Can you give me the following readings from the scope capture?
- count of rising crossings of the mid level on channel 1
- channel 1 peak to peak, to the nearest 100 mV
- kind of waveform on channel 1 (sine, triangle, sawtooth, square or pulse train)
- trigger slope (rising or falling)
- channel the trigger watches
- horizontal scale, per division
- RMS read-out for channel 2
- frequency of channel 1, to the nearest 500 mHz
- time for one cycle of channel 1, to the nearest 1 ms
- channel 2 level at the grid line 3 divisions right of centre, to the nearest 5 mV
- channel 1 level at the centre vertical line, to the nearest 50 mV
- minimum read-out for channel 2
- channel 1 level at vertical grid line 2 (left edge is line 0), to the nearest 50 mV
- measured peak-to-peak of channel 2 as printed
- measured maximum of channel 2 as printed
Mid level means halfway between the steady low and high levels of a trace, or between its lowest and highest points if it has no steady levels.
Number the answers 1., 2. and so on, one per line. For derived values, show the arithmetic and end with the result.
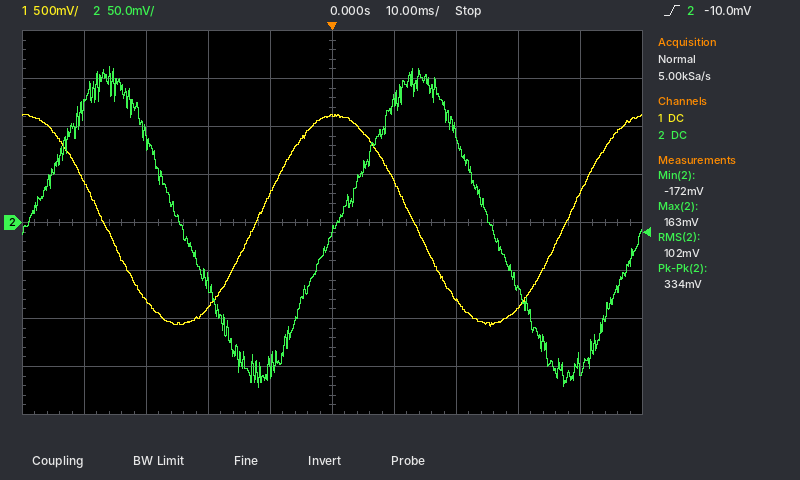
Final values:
1. 2
2. 2.20 V
3. sine
4. rising
5. channel 2
6. 10 ms
7. 102 mV
8. 1 / 50 ms ≈ 20.0 Hz
9. 50 ms
10. -70 mV
11. 1.10 V
12. -172 mV
13. -800 mV
14. 334 mV
15. 163 mV
